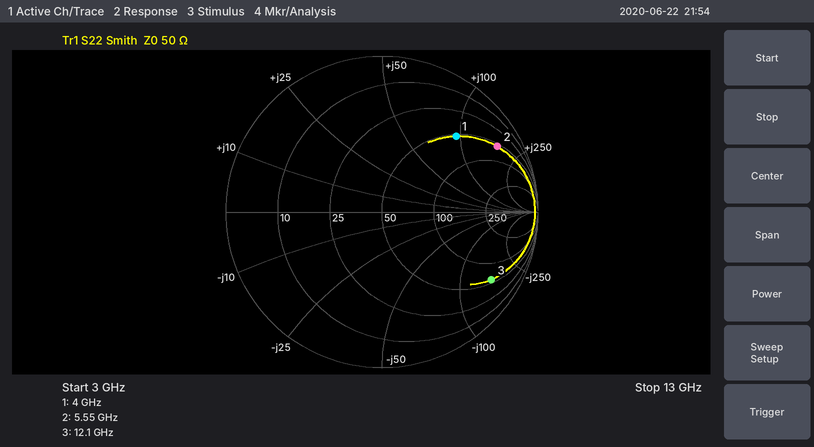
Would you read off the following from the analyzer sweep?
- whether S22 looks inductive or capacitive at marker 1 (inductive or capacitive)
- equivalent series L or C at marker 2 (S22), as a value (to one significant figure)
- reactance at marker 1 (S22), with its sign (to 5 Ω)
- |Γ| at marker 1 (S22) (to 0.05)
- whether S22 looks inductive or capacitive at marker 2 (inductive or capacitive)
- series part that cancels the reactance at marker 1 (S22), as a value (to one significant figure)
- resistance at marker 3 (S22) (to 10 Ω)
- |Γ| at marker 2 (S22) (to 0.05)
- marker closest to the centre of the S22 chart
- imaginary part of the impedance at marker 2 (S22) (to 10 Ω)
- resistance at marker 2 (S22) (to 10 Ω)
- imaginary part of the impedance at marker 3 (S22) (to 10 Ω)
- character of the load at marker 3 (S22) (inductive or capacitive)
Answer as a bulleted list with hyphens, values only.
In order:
- inductive
- 5 nH
- +95 Ω
- 0.70
- inductive
- 400 fF
- 60 Ω
- 0.85
- marker 1
- +170 Ω
- 60 Ω
- -160 Ω
- capacitive
